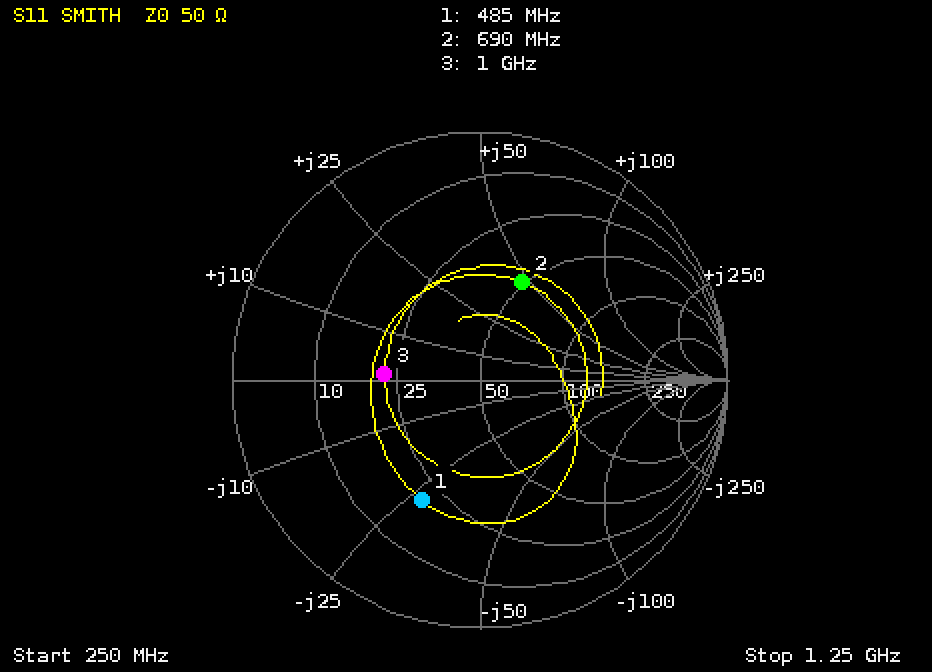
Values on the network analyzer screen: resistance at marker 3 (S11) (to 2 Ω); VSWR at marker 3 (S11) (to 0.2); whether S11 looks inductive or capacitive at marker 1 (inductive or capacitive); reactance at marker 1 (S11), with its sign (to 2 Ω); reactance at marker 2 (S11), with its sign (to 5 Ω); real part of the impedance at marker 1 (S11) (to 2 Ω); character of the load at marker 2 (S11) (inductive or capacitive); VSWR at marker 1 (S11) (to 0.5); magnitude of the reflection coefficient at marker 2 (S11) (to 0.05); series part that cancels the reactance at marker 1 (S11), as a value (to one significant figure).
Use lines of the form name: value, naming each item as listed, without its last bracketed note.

resistance at marker 3 (S11): 22 Ω
VSWR at marker 3 (S11): 2.2
whether S11 looks inductive or capacitive at marker 1: capacitive
reactance at marker 1 (S11), with its sign: -28 Ω
reactance at marker 2 (S11), with its sign: +45 Ω
real part of the impedance at marker 1 (S11): 20 Ω
character of the load at marker 2 (S11): inductive
VSWR at marker 1 (S11): 3.5
magnitude of the reflection coefficient at marker 2 (S11): 0.45
series part that cancels the reactance at marker 1 (S11), as a value: 9 nH
